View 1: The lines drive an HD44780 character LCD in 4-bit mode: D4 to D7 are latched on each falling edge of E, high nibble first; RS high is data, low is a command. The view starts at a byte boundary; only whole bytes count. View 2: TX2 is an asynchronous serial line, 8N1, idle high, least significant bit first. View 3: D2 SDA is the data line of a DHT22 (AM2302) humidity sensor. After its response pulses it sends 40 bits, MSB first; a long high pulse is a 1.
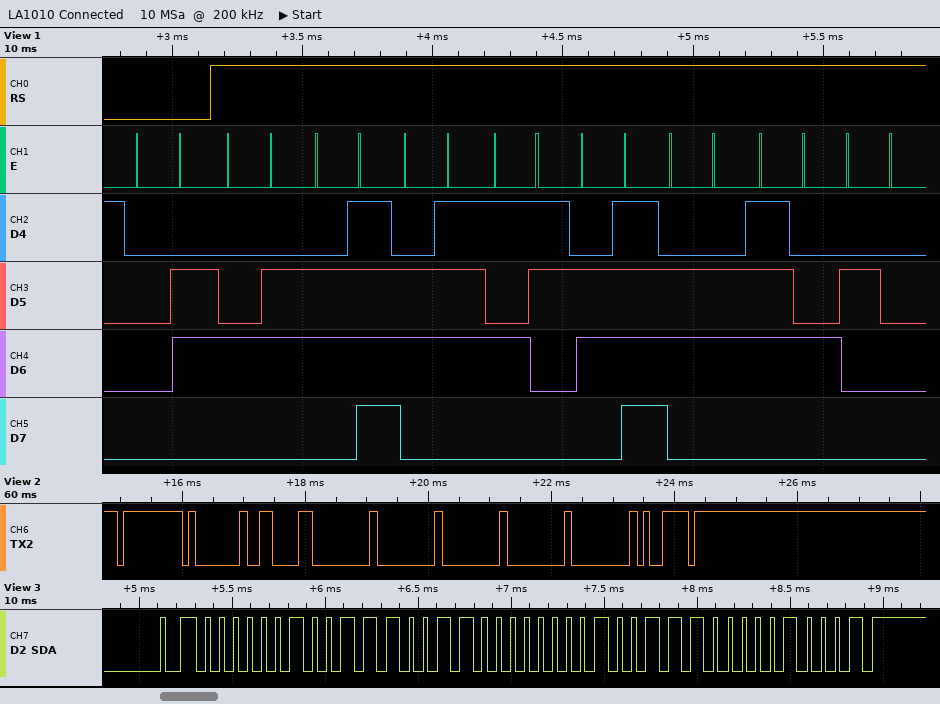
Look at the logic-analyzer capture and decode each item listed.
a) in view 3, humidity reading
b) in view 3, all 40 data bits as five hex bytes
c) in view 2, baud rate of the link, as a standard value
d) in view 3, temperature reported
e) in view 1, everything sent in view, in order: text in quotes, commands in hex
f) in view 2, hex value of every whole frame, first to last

62.7 %
02 73 00 9C 11
9600 baud
15.6 °C
0x06 "FogSoft "
FF 01 86 00 00 00 00 00 79
